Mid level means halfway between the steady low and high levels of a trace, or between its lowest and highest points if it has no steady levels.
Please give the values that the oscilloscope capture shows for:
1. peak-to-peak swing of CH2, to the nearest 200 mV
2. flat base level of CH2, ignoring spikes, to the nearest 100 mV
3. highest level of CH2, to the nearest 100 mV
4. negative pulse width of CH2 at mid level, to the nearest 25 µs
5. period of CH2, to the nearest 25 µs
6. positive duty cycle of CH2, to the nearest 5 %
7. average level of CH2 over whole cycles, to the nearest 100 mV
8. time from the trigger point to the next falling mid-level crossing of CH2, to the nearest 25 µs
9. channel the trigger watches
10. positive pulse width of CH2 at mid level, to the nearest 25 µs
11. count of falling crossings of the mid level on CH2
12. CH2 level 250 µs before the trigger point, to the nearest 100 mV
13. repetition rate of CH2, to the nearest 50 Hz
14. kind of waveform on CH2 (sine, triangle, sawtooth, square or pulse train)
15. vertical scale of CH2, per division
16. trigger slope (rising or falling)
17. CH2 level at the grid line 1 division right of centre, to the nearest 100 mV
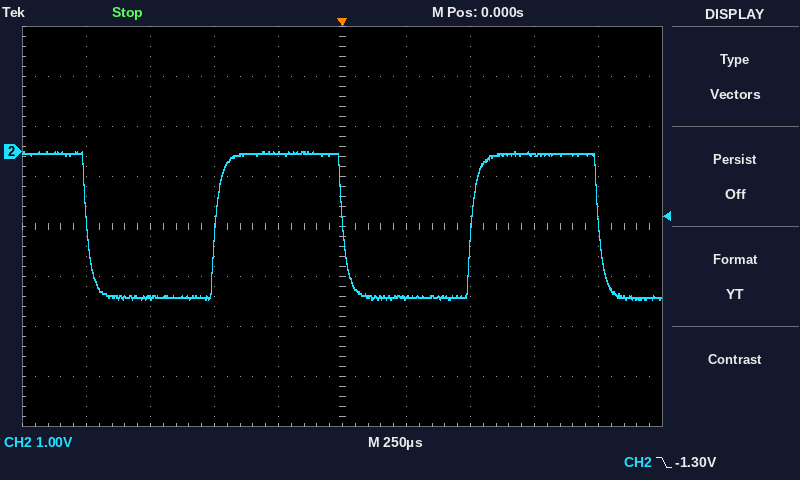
3.0 V
-2.9 V
0.0 V
500 µs
1.000 ms
50 %
-1.5 V
1.000 ms
CH2
500 µs
3
0.0 V
1.00 kHz
square
1 V
falling
-2.9 V
